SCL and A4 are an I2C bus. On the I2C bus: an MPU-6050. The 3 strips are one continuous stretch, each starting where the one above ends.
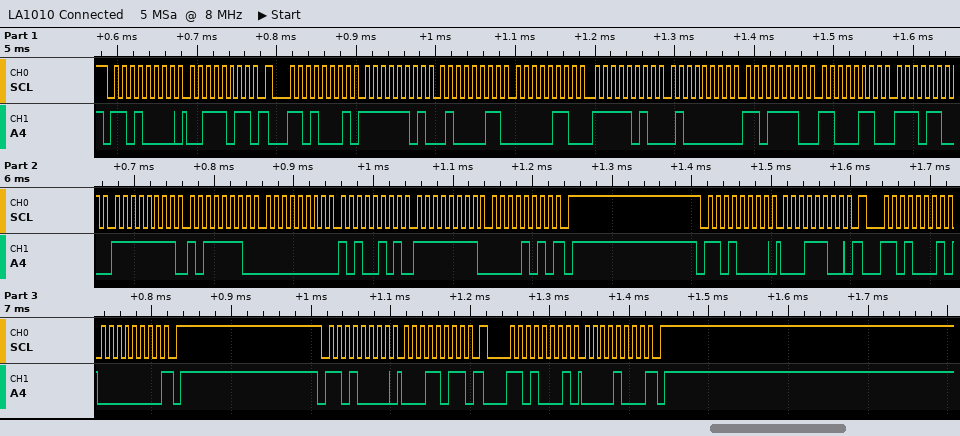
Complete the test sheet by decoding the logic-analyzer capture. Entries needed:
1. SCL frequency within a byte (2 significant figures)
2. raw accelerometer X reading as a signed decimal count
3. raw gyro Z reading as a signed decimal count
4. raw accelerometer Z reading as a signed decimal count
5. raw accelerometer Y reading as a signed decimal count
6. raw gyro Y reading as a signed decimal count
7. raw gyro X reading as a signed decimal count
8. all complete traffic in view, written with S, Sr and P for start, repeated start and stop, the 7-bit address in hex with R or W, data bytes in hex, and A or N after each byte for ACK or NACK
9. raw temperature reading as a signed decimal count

100 kHz
-701
-246
16606
1786
165
-66
S 68W A 3B A Sr 68R A FD A 43 A 06 A FA A 40 A DE A C6 A EC A FF A BE A 00 A A5 A FF A 0A N P S 68W A 1C A Sr 68R A 00 N P S 68W A 1B A Sr 68R A 08 N P
-14612
